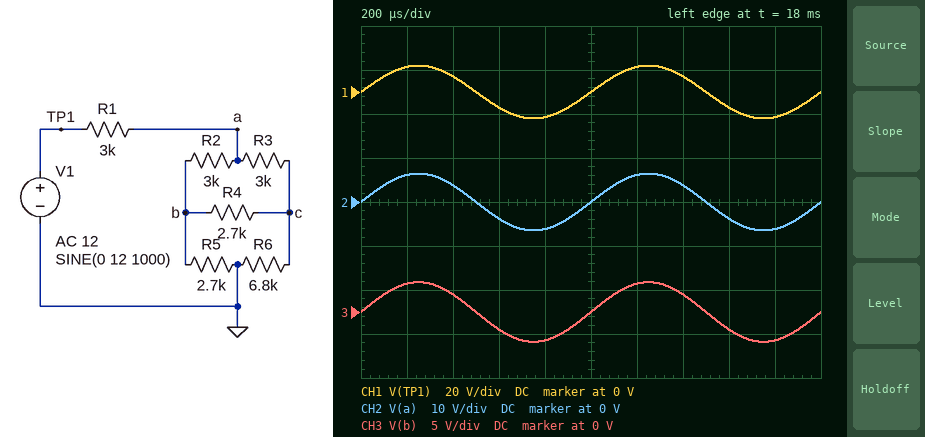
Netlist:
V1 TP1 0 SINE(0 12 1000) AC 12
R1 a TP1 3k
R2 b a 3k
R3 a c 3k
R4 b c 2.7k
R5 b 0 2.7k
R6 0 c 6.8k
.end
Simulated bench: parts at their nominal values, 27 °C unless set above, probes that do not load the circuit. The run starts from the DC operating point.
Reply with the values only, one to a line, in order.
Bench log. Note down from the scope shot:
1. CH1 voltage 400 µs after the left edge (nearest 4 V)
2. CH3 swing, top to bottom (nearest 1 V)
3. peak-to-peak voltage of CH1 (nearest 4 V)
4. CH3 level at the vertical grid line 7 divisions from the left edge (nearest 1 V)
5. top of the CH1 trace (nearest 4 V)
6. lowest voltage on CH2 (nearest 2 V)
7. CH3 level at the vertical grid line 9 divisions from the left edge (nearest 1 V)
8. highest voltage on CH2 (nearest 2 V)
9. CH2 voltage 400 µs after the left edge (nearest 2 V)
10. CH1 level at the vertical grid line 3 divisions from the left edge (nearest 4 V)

8 V
7 V
24 V
2 V
12 V
-6 V
-3 V
6 V
4 V
-8 V
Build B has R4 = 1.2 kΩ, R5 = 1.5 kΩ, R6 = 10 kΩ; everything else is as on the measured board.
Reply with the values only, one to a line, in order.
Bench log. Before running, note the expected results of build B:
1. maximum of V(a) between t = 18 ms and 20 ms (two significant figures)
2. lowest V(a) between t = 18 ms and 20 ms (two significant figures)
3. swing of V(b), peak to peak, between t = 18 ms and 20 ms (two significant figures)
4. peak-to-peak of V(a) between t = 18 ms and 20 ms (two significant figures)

5.9 V
-5.9 V
5.1 V
12 V
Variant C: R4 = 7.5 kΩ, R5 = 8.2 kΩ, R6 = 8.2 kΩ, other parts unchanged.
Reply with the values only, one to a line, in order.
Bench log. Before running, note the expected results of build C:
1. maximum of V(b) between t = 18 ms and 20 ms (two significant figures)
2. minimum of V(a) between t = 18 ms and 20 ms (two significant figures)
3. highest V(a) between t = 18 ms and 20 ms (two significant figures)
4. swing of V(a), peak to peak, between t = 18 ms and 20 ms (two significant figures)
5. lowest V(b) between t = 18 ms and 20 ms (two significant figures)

5.7 V
-7.8 V
7.8 V
16 V
-5.7 V
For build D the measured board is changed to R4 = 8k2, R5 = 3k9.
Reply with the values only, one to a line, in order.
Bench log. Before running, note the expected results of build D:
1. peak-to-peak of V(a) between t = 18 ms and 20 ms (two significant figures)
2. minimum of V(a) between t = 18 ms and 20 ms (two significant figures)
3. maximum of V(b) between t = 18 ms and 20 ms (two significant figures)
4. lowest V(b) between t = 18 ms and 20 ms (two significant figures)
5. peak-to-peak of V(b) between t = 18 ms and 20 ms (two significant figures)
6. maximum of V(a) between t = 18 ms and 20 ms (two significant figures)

14 V
-6.9 V
4.0 V
-4.0 V
8.0 V
6.9 V
